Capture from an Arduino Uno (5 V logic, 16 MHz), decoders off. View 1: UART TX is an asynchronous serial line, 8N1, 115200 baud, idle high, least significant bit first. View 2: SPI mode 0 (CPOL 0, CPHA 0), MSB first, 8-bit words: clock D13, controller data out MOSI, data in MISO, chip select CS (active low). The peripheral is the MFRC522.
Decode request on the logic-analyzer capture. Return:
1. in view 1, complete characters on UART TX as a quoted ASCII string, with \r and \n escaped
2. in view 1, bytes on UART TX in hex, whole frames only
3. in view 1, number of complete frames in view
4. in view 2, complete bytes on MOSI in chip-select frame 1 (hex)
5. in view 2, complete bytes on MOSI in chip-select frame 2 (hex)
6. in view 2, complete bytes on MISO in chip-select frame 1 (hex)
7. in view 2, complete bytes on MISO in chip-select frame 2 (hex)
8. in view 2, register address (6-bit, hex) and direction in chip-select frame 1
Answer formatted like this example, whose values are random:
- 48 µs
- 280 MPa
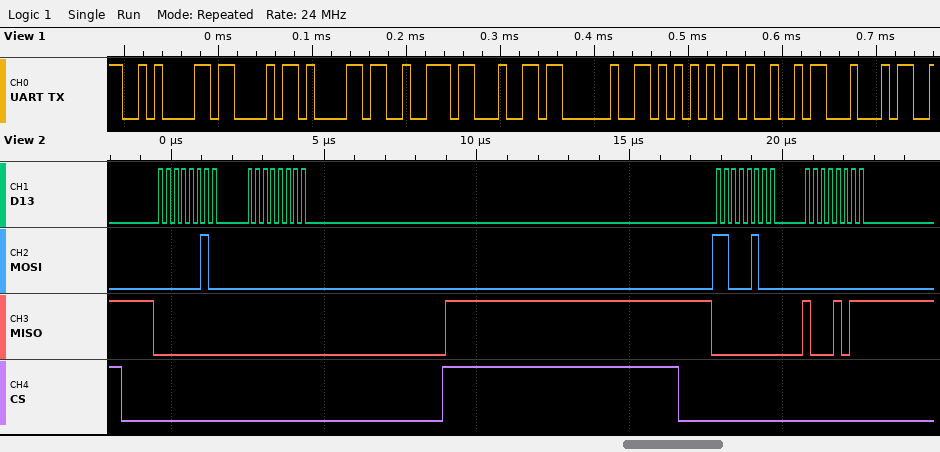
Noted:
- "\nCard UID"
- 0A 43 61 72 64 20 55 49 44
- 9
- 0x02 0x00
- 0xC4 0x00
- 0x00 0x00
- 0x00 0x8B
- 0x01 write
